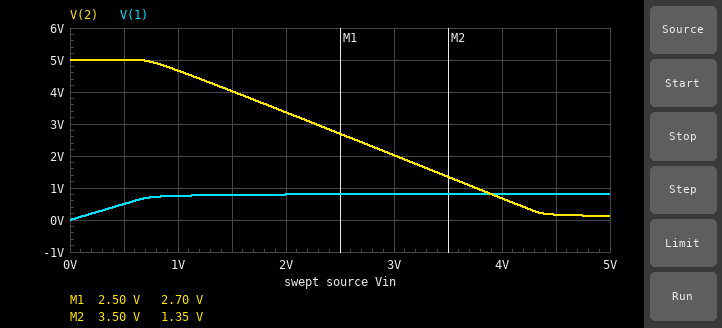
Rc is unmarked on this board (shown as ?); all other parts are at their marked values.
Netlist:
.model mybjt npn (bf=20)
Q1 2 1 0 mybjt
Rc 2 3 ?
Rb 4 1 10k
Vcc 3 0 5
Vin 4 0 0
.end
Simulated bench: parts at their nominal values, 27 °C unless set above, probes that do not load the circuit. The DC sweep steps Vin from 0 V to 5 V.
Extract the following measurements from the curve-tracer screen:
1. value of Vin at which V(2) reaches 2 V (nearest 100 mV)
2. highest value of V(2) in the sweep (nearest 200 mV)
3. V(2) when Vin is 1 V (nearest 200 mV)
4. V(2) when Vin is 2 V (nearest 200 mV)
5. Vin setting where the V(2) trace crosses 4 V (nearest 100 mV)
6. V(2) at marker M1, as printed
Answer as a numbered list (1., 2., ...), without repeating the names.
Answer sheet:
1. 3.0 V
2. 5.0 V
3. 4.6 V
4. 3.4 V
5. 1.5 V
6. 2.70 V
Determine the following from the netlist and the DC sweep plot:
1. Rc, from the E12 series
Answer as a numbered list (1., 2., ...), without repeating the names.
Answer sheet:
1. 680 Ω
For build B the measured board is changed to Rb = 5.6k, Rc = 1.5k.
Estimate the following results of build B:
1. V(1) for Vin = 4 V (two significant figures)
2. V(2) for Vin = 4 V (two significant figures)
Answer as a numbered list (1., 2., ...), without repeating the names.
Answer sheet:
1. 810 mV
2. 62 mV
